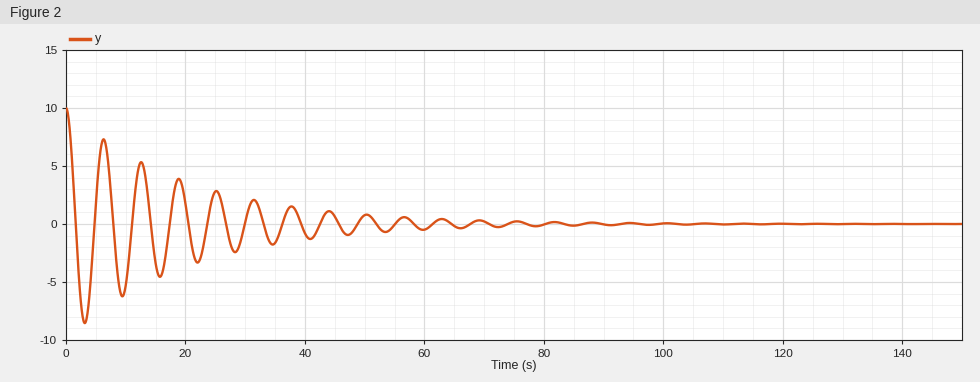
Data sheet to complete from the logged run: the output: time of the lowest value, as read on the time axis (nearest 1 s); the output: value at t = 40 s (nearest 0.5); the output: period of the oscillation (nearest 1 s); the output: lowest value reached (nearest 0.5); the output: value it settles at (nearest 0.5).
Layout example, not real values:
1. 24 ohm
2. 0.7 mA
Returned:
1. 3 s
2. -1.0
3. 6 s
4. -8.5
5. 0.0
